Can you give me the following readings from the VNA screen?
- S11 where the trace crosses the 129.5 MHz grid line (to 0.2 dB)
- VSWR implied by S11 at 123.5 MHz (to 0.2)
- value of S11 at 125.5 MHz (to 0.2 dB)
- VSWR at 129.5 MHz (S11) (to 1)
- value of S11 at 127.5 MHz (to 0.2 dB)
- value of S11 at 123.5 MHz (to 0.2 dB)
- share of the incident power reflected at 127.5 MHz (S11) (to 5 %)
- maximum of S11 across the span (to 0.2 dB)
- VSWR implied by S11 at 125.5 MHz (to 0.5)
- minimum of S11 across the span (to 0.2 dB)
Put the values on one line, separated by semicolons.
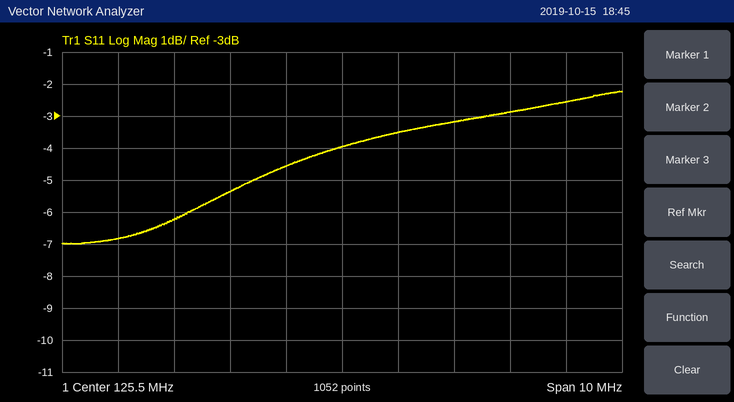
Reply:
-2.6 dB; 3.4; -4.0 dB; 7; -3.2 dB; -5.4 dB; 50 %; -2.2 dB; 4.5; -7.0 dB
